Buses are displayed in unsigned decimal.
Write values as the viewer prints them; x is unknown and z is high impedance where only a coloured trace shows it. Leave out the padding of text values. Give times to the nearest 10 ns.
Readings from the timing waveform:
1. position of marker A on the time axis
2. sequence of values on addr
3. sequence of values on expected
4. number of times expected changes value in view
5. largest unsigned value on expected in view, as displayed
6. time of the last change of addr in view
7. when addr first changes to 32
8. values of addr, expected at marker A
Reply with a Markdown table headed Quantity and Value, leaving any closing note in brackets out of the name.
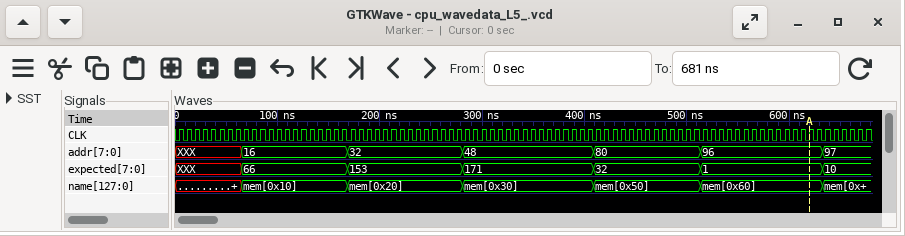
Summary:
| Quantity | Value |
|---|---|
| position of marker A on the time axis | 620 ns |
| sequence of values on addr | XXX, 16, 32, 48, 80, 96, 97 |
| sequence of values on expected | XXX, 66, 153, 171, 32, 1, 10 |
| number of times expected changes value in view | 6 |
| largest unsigned value on expected in view, as displayed | 171 |
| time of the last change of addr in view | 630 ns |
| when addr first changes to 32 | 170 ns |
| values of addr, expected at marker A | addr=96, expected=1 |
